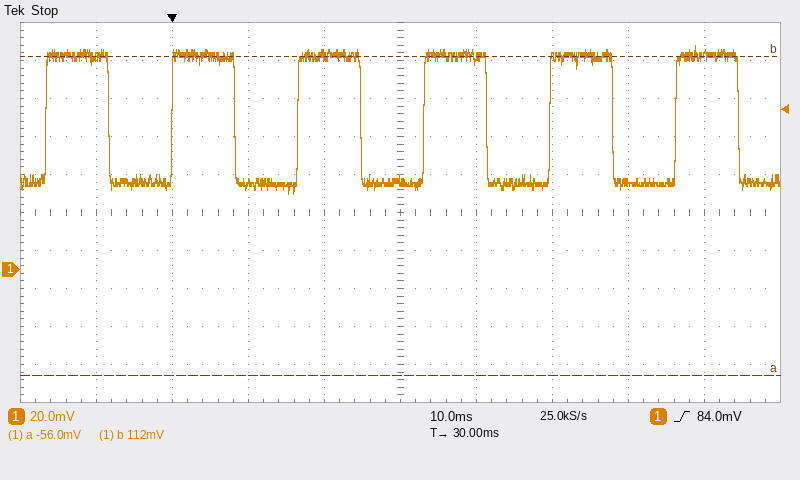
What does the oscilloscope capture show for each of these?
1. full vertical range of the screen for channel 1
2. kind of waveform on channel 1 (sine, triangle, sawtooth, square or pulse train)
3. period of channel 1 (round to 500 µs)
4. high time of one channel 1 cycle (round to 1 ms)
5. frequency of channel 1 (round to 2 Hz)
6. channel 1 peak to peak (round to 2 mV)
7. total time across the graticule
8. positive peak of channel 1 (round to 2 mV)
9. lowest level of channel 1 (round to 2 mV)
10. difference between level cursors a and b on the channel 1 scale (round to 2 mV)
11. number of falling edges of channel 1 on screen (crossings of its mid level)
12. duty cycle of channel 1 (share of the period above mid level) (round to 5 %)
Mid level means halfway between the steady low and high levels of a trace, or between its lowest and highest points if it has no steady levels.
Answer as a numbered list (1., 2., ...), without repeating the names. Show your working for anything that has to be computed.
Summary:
1. 200 mV
2. square
3. 16.5 ms
4. 8 ms
5. 1 / 16.5 ms ≈ 60.6 Hz, so 60 Hz to the nearest 2 Hz
6. 118 mV − (40 mV) = 78 mV
7. 100 ms
8. 118 mV
9. 40 mV
10. 168 mV
11. 6
12. 8 ms / 16.5 ms ≈ 48.5 %, so 50 % to the nearest 5 %
